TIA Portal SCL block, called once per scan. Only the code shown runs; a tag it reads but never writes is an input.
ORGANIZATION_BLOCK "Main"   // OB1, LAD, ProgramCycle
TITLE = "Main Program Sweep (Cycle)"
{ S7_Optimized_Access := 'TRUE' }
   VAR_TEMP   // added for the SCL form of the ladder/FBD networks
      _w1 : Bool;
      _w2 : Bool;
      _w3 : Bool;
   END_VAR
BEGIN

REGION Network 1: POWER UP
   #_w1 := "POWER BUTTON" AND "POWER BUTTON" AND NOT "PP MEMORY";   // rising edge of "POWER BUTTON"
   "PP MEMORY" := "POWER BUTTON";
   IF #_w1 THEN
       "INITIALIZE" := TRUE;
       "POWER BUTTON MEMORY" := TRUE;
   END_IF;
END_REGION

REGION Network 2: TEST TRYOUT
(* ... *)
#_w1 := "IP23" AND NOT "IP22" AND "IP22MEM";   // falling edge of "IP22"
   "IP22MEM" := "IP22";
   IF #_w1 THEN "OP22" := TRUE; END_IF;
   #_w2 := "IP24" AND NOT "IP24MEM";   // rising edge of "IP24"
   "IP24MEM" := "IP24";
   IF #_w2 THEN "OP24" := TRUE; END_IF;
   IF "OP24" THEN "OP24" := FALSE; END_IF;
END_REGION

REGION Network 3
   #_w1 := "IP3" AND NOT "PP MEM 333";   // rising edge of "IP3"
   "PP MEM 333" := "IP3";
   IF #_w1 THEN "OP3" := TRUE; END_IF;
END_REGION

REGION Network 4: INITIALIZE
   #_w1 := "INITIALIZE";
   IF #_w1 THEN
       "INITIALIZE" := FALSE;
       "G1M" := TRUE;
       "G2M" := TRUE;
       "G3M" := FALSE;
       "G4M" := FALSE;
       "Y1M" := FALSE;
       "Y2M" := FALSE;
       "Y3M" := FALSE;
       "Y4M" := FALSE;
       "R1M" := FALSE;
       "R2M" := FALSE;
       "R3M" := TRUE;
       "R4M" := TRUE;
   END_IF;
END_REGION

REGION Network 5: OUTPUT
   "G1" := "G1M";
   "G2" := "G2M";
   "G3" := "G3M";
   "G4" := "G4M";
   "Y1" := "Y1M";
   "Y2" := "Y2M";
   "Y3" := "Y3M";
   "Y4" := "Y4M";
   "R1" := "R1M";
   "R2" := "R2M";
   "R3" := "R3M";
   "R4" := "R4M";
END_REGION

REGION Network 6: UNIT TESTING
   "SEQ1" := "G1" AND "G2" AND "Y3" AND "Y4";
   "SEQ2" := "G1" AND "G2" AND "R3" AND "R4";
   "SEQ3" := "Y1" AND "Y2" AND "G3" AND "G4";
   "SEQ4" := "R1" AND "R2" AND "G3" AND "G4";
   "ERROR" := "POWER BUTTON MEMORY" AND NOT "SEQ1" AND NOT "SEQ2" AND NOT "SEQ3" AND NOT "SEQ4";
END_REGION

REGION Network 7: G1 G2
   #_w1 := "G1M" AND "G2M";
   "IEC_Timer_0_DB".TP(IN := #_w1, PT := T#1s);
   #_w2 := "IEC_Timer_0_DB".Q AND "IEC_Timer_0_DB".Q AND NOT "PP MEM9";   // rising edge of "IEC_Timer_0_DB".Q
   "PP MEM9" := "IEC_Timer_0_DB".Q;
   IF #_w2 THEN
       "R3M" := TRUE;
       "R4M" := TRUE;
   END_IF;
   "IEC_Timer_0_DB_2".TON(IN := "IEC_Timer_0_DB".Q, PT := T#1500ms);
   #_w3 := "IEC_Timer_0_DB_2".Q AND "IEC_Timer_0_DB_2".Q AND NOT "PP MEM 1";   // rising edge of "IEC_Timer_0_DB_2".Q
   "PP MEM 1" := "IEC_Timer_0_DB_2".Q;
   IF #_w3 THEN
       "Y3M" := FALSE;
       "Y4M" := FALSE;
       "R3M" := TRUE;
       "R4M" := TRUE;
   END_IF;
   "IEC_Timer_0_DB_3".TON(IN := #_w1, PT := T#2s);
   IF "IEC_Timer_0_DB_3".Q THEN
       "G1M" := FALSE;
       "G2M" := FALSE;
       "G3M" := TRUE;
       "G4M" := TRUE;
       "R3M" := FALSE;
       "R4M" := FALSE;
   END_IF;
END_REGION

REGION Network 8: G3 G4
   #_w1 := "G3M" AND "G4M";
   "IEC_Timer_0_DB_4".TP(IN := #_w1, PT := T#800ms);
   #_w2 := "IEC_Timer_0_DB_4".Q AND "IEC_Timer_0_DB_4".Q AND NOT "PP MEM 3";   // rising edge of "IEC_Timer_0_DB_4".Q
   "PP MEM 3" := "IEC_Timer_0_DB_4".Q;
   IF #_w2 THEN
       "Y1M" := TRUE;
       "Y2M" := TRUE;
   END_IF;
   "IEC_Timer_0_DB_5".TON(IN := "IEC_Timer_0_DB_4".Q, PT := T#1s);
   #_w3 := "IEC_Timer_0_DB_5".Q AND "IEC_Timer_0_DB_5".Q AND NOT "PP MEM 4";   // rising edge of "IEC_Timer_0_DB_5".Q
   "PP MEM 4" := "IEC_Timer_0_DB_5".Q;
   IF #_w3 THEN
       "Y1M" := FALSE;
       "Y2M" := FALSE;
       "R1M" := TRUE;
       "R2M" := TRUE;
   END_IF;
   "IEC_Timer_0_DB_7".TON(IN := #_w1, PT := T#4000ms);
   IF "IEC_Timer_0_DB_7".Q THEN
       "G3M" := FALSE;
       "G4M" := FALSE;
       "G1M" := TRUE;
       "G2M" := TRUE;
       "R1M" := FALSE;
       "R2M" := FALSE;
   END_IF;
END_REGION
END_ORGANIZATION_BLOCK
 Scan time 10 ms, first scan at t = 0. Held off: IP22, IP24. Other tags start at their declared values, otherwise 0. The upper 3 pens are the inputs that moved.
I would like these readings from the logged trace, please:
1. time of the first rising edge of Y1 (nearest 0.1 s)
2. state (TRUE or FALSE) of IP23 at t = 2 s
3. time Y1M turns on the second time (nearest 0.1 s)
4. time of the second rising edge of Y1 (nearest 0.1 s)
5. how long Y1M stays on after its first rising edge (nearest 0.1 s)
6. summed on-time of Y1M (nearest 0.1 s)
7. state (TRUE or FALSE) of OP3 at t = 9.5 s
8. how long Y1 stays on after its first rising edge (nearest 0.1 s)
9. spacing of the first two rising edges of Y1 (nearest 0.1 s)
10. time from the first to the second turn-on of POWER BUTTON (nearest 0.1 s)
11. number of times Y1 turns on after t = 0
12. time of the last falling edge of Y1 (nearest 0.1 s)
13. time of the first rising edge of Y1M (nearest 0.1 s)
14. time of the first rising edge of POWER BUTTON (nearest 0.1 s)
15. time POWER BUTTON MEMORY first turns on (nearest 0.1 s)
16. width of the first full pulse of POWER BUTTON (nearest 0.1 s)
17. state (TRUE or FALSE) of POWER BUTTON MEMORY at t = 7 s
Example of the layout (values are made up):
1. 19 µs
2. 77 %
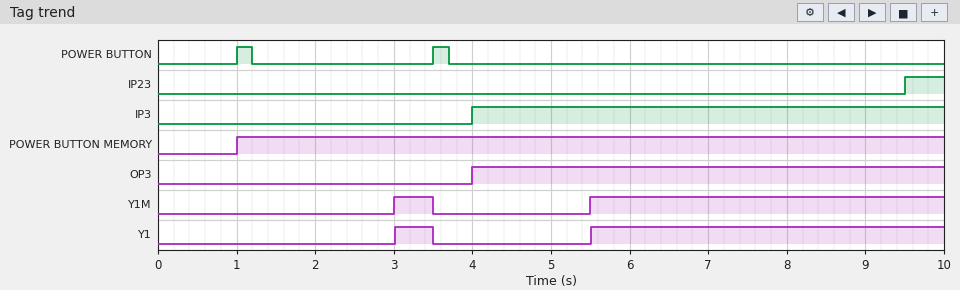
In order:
1. 3.0 s
2. FALSE
3. 5.5 s
4. 5.5 s
5. 0.5 s
6. 5.0 s
7. TRUE
8. 0.5 s
9. 2.5 s
10. 2.5 s
11. 2
12. 3.5 s
13. 3.0 s
14. 1.0 s
15. 1.0 s
16. 0.2 s
17. TRUE
